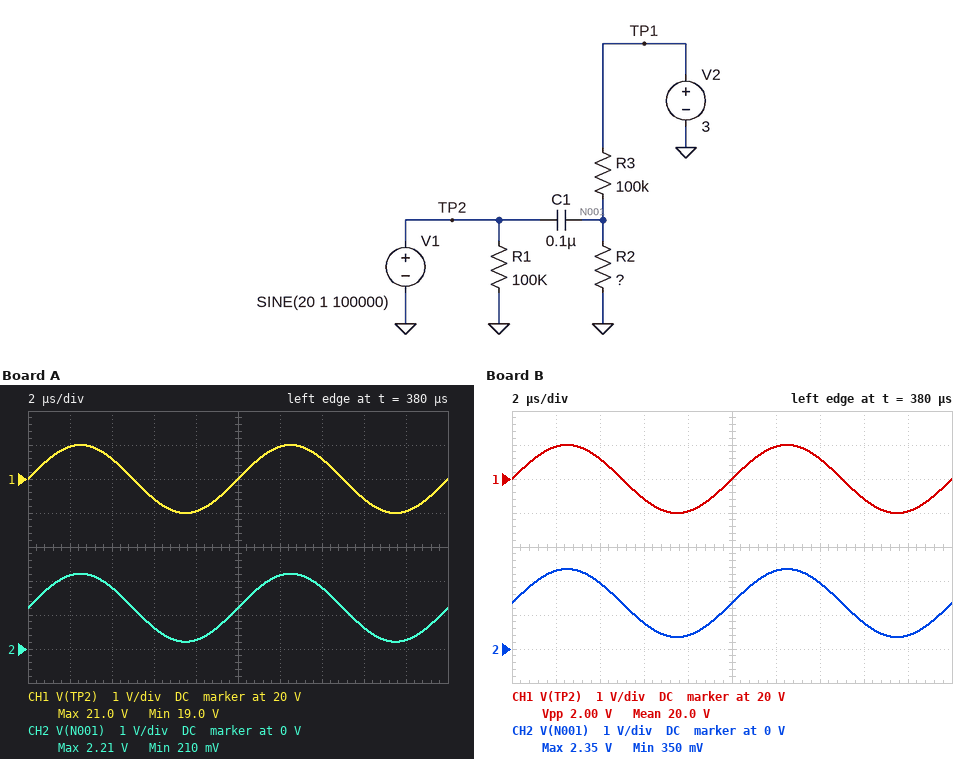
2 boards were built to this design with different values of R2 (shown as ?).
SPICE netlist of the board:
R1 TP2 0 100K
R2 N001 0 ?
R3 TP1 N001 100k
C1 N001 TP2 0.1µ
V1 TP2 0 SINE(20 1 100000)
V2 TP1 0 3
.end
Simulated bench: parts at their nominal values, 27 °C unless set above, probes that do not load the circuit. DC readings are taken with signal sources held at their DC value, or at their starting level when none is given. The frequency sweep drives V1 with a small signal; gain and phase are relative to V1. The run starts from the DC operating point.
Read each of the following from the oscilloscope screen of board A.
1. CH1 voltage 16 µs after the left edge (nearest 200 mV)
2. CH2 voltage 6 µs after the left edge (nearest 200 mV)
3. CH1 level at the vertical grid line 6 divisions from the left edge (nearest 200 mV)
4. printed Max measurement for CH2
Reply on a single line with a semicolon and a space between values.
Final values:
19.4 V; 600 mV; 21.0 V; 2.21 V
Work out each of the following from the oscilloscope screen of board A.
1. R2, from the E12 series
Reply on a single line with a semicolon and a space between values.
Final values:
68 kΩ
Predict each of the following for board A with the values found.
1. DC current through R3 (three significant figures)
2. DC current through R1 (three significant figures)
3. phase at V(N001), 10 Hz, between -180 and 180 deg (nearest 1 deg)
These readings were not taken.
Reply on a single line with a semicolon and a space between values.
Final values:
17.9 µA; 200 µA; 76 deg
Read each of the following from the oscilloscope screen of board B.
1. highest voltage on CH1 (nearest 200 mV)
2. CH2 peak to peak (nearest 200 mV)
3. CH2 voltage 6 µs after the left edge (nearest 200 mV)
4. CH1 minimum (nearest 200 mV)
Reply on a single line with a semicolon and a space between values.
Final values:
21.0 V; 2.0 V; 800 mV; 19.0 V
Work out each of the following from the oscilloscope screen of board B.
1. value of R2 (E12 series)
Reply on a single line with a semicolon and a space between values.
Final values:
82 kΩ
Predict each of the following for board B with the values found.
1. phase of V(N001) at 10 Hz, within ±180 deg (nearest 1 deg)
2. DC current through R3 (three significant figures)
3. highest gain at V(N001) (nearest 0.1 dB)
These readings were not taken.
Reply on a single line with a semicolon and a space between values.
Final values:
74 deg; 16.5 µA; 0 dB
